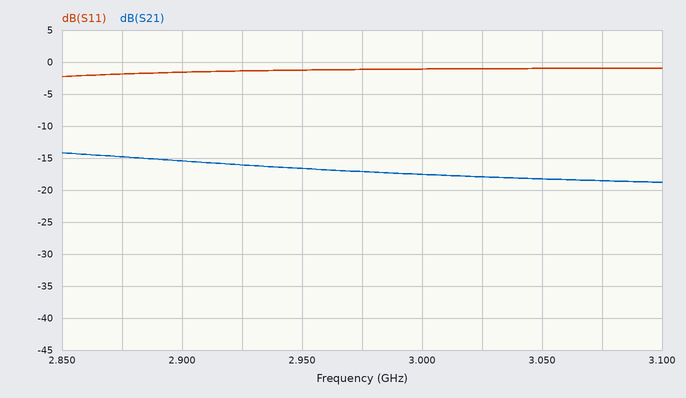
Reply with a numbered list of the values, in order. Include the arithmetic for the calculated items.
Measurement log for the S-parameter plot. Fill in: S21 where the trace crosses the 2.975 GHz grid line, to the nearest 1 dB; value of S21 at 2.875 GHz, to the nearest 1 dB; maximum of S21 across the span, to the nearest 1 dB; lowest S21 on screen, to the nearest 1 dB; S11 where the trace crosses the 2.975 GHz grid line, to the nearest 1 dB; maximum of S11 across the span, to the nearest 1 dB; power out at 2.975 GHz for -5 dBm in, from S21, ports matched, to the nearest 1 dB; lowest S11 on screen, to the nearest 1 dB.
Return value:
1. -17 dB
2. -15 dB
3. -14 dB
4. -19 dB
5. -1 dB
6. -1 dB
7. -5 dBm + (-17 dB) = -22 dBm
8. -2 dB
